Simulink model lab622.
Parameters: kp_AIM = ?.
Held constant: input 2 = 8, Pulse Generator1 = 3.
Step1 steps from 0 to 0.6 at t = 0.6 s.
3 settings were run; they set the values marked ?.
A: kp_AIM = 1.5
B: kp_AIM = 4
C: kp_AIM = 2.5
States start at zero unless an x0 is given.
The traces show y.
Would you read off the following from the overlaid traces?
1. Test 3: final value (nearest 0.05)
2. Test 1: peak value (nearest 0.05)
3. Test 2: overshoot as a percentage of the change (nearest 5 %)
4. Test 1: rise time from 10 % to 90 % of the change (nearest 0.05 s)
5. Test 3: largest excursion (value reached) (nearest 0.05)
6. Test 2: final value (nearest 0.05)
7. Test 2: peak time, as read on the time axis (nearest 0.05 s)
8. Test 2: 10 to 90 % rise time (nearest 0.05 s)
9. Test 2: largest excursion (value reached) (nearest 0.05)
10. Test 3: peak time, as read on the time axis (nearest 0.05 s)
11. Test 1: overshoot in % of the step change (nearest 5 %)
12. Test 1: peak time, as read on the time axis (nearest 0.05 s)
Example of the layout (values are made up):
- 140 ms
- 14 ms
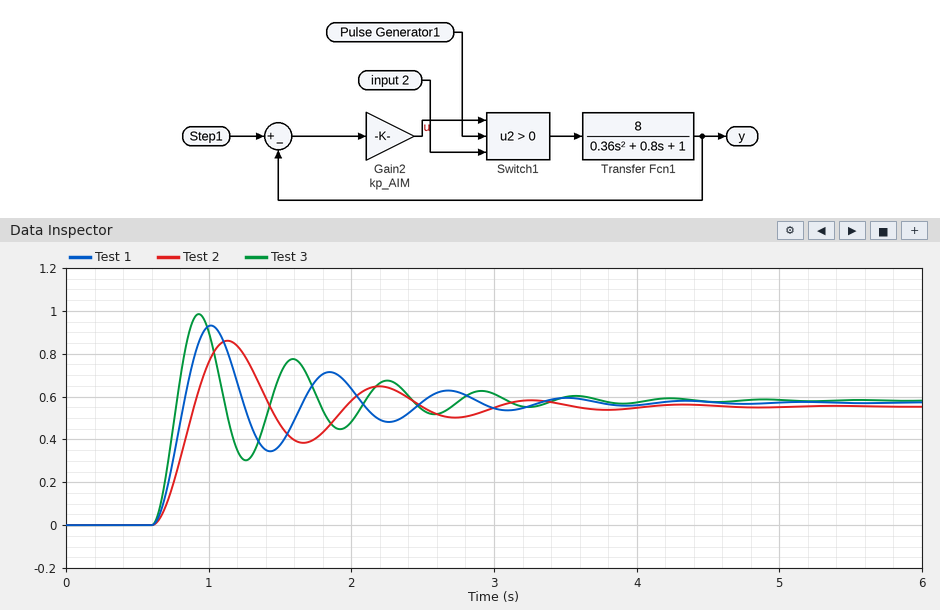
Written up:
- 0.60
- 0.95
- 55 %
- 0.15 s
- 1.00
- 0.55
- 1.15 s
- 0.20 s
- 0.85
- 0.95 s
- 65 %
- 1.00 s
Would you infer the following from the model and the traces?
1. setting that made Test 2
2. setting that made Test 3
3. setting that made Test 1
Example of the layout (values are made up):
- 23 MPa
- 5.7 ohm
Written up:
- A
- B
- C
